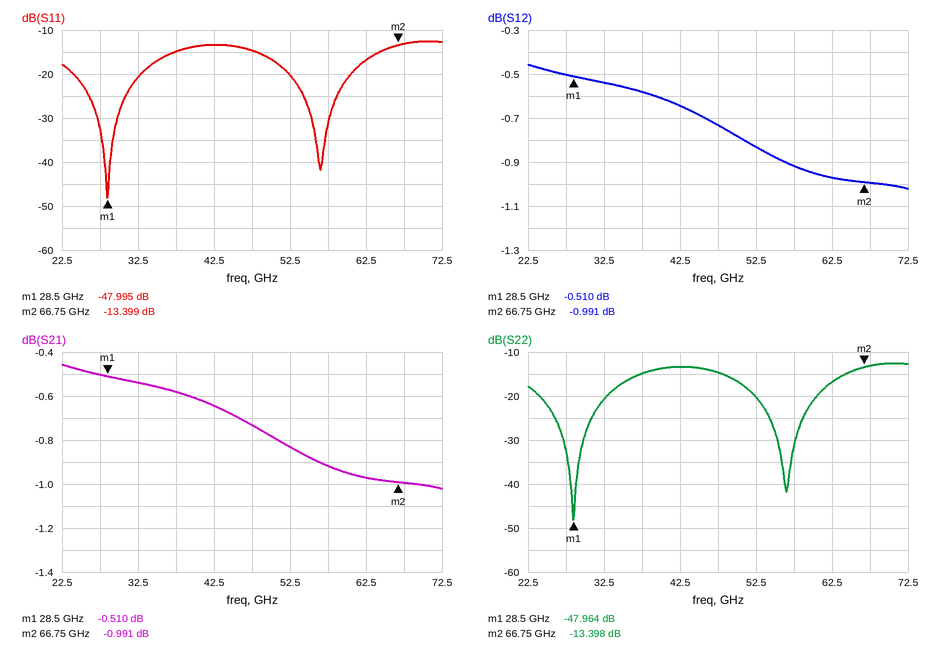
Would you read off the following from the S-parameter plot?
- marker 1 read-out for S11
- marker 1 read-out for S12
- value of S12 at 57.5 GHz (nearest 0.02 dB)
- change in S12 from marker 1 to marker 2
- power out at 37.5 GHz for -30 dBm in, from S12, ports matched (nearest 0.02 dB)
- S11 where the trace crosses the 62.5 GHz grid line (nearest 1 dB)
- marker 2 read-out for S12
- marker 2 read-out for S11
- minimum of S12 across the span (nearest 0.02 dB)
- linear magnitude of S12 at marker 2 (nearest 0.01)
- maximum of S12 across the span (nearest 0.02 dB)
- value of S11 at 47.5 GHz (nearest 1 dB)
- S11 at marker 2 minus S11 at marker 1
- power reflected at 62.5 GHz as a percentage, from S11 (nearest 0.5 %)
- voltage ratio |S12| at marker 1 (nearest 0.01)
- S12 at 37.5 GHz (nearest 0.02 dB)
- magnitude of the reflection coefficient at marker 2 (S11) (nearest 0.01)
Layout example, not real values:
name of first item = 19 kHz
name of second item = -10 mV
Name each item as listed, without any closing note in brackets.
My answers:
marker 1 read-out for S11 = -47.995 dB
marker 1 read-out for S12 = -0.510 dB
value of S12 at 57.5 GHz = -0.92 dB
change in S12 from marker 1 to marker 2 = -0.481 dB
power out at 37.5 GHz for -30 dBm in, from S12, ports matched = -30.58 dBm
S11 where the trace crosses the 62.5 GHz grid line = -17 dB
marker 2 read-out for S12 = -0.991 dB
marker 2 read-out for S11 = -13.399 dB
minimum of S12 across the span = -1.02 dB
linear magnitude of S12 at marker 2 = 0.89
maximum of S12 across the span = -0.46 dB
value of S11 at 47.5 GHz = -15 dB
S11 at marker 2 minus S11 at marker 1 = 34.596 dB
power reflected at 62.5 GHz as a percentage, from S11 = 2.0 %
voltage ratio |S12| at marker 1 = 0.94
S12 at 37.5 GHz = -0.58 dB
magnitude of the reflection coefficient at marker 2 (S11) = 0.21
